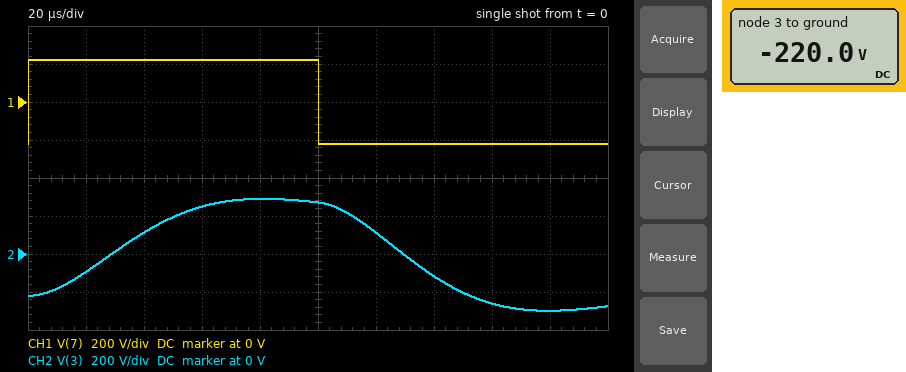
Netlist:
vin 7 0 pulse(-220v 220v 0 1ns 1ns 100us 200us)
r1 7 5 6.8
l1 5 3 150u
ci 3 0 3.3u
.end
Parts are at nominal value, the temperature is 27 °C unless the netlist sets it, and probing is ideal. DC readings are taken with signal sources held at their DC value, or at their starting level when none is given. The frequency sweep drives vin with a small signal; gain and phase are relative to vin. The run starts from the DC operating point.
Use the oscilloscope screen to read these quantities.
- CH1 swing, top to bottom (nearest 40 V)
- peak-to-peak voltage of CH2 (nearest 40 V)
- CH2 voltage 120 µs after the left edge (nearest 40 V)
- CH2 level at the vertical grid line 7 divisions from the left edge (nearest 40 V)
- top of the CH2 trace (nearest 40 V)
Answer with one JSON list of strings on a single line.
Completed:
["440 V", "600 V", "120 V", "-120 V", "280 V"]
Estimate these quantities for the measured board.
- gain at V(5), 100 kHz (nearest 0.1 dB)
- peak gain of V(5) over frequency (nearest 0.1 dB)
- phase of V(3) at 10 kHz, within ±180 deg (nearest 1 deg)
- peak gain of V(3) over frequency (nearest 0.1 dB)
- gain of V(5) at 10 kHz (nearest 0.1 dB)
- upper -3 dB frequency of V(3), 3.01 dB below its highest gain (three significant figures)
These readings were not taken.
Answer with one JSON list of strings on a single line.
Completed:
["0 dB", "0 dB", "-124 deg", "1.2 dB", "-5.0 dB", "8.35 kHz"]
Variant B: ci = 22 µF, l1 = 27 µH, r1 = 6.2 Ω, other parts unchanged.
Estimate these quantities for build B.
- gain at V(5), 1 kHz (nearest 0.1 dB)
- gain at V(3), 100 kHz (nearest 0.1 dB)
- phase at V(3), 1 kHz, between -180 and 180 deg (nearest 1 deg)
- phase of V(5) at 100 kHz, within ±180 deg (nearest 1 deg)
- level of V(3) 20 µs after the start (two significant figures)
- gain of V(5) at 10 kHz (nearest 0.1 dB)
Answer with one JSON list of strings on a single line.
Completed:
["-2.5 dB", "-47.9 dB", "-41 deg", "20 deg", "-170 V", "-16.2 dB"]
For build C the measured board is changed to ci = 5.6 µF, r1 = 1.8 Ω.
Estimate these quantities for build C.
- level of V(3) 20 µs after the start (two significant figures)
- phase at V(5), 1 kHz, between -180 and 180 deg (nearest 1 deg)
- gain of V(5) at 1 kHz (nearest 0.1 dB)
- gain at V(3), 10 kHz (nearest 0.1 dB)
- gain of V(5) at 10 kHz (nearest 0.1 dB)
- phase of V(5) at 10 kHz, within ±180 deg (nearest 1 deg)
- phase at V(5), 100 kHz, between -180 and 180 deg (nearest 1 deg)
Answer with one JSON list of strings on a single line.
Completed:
["-130 V", "-4 deg", "0 dB", "-7.6 dB", "-0.3 dB", "15 deg", "1 deg"]
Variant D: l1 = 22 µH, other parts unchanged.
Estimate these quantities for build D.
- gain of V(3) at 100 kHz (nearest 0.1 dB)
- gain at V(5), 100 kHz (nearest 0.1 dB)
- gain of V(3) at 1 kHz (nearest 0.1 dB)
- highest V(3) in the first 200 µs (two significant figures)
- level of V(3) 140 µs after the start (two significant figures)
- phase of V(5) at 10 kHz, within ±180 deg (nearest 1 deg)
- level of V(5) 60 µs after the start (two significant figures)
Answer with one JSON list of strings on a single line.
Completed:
["-29.8 dB", "-1.0 dB", "-0.1 dB", "220 V", "-160 V", "-63 deg", "190 V"]
